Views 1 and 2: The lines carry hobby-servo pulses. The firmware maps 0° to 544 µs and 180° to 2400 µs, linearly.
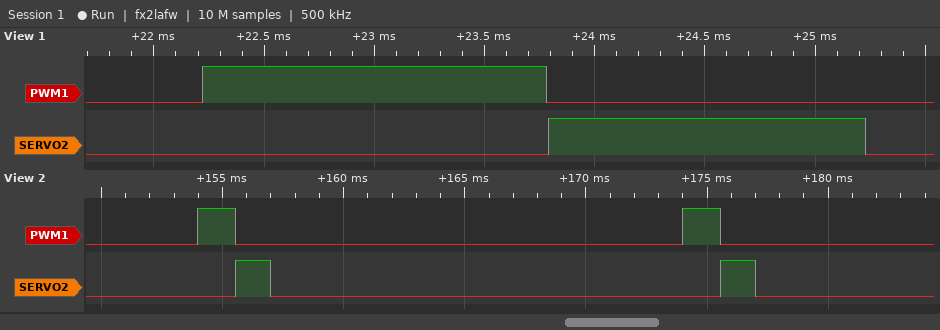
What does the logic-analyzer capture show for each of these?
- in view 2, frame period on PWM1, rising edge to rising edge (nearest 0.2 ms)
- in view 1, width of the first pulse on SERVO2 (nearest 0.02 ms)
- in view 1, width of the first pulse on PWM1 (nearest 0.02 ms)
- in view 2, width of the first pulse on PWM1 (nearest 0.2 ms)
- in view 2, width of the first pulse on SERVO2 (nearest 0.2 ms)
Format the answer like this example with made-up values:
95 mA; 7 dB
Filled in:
20.0 ms; 1.44 ms; 1.56 ms; 1.6 ms; 1.4 ms
